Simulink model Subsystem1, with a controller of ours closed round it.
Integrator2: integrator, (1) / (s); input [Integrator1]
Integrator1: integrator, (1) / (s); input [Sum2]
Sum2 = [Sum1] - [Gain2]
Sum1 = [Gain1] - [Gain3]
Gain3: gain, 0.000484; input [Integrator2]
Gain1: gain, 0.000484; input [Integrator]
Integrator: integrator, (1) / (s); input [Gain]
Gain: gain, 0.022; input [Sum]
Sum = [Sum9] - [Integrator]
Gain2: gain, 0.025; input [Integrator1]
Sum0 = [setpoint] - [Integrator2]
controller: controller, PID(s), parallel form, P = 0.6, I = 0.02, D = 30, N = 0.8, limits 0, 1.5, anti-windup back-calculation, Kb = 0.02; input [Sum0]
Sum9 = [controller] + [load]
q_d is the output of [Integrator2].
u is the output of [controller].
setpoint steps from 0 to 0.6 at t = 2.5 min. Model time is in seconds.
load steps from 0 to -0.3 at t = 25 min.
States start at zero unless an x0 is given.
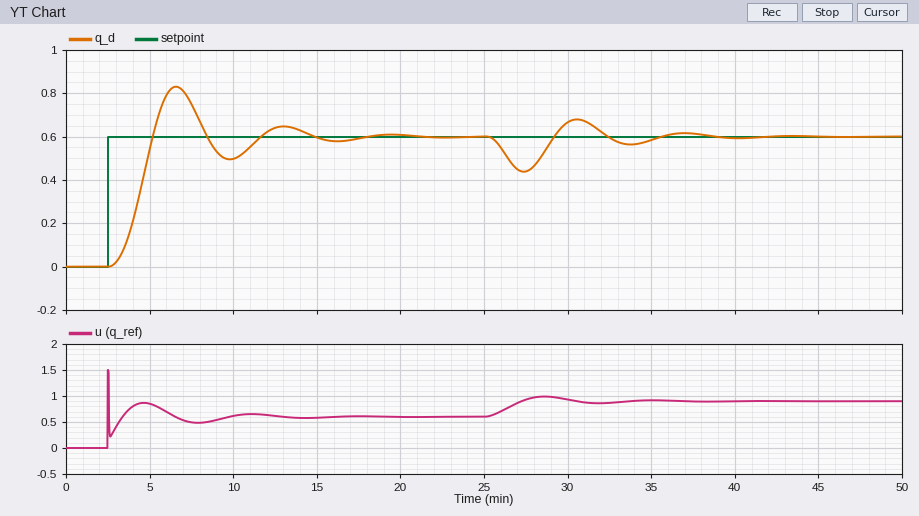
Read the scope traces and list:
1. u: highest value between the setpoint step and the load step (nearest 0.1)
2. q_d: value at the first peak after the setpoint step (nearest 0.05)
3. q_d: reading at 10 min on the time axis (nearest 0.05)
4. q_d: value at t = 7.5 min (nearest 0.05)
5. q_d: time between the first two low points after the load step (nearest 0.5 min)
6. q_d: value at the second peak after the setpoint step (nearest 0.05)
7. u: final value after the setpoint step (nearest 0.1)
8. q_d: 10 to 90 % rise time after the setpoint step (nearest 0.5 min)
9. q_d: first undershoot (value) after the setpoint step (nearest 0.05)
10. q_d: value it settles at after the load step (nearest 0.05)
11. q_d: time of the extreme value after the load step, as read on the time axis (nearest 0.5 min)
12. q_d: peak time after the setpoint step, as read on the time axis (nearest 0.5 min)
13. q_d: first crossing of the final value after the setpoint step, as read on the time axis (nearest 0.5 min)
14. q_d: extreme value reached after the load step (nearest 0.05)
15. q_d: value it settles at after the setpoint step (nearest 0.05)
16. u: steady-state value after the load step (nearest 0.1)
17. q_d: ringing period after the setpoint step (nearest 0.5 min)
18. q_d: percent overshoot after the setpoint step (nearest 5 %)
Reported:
1.5
0.85
0.50
0.75
6.5 min
0.65
0.6
1.5 min
0.50
0.60
27.5 min
6.5 min
5.0 min
0.45
0.60
0.9
6.5 min
40 %
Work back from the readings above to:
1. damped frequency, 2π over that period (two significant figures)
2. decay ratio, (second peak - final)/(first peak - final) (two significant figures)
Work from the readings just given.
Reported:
0.97 rad/min
0.20
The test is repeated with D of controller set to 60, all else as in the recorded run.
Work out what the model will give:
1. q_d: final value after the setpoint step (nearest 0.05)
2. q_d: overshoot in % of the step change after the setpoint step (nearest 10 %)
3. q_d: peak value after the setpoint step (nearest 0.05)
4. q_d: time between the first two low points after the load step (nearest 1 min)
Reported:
0.60
30 %
0.80
8 min
